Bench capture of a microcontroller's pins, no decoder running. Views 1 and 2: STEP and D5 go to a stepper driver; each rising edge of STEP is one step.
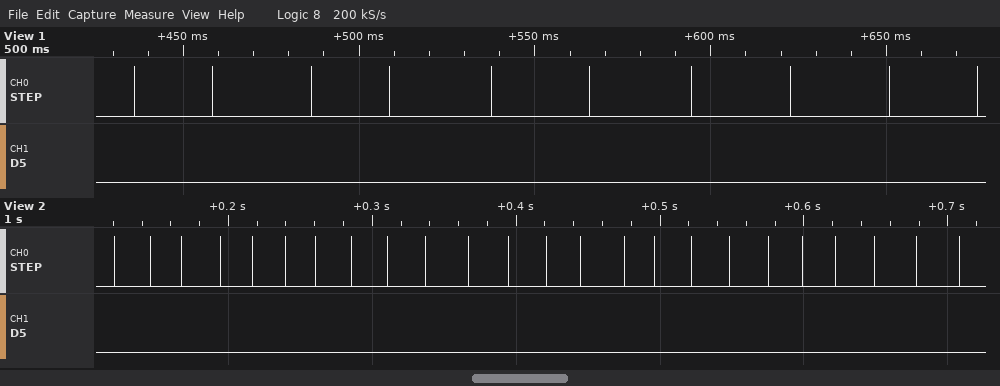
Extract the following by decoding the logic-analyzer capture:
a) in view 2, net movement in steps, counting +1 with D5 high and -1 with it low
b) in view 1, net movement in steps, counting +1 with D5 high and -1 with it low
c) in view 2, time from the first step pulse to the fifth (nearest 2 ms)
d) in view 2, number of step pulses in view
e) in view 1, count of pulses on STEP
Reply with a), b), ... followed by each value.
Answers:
a) -24
b) -10
c) 96 ms
d) 24
e) 10
